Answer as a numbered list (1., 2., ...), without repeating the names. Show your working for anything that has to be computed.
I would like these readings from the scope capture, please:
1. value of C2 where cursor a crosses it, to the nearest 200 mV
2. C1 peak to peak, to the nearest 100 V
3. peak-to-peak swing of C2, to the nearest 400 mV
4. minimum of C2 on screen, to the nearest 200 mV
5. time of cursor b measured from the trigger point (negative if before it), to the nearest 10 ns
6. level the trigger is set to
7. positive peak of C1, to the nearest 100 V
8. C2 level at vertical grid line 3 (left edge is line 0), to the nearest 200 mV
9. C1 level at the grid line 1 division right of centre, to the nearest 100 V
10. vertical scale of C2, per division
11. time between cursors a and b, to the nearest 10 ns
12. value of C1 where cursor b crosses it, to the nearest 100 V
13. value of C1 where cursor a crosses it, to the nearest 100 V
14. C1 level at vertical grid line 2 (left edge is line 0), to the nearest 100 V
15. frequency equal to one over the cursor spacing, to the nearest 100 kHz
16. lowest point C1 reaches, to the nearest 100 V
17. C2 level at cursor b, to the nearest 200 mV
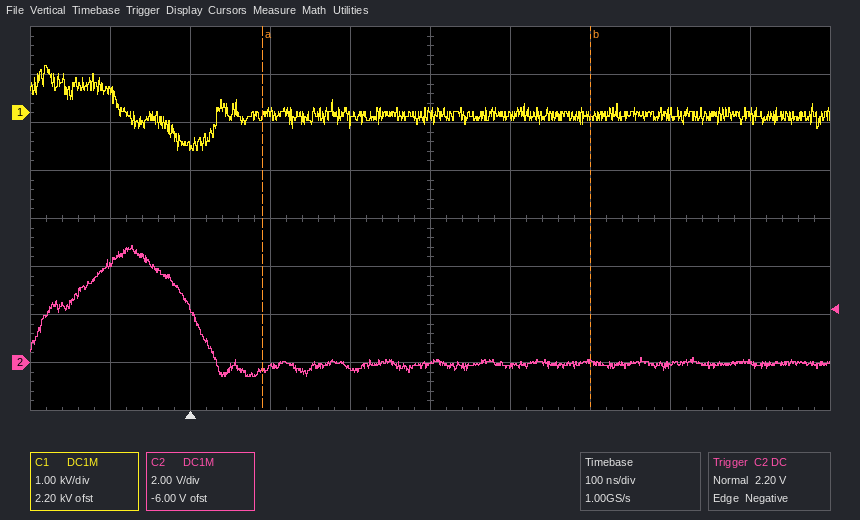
1. -400 mV
2. 1.0 kV − (-800 V) = 1.8 kV
3. 5.6 V
4. -600 mV
5. +500 ns
6. 2.20 V
7. 1.0 kV
8. -200 mV
9. -100 V
10. 2 V
11. 410 ns
12. -100 V
13. -100 V
14. -700 V
15. 1 / 410 ns ≈ 2.4 MHz
16. -800 V
17. 0.0 V
